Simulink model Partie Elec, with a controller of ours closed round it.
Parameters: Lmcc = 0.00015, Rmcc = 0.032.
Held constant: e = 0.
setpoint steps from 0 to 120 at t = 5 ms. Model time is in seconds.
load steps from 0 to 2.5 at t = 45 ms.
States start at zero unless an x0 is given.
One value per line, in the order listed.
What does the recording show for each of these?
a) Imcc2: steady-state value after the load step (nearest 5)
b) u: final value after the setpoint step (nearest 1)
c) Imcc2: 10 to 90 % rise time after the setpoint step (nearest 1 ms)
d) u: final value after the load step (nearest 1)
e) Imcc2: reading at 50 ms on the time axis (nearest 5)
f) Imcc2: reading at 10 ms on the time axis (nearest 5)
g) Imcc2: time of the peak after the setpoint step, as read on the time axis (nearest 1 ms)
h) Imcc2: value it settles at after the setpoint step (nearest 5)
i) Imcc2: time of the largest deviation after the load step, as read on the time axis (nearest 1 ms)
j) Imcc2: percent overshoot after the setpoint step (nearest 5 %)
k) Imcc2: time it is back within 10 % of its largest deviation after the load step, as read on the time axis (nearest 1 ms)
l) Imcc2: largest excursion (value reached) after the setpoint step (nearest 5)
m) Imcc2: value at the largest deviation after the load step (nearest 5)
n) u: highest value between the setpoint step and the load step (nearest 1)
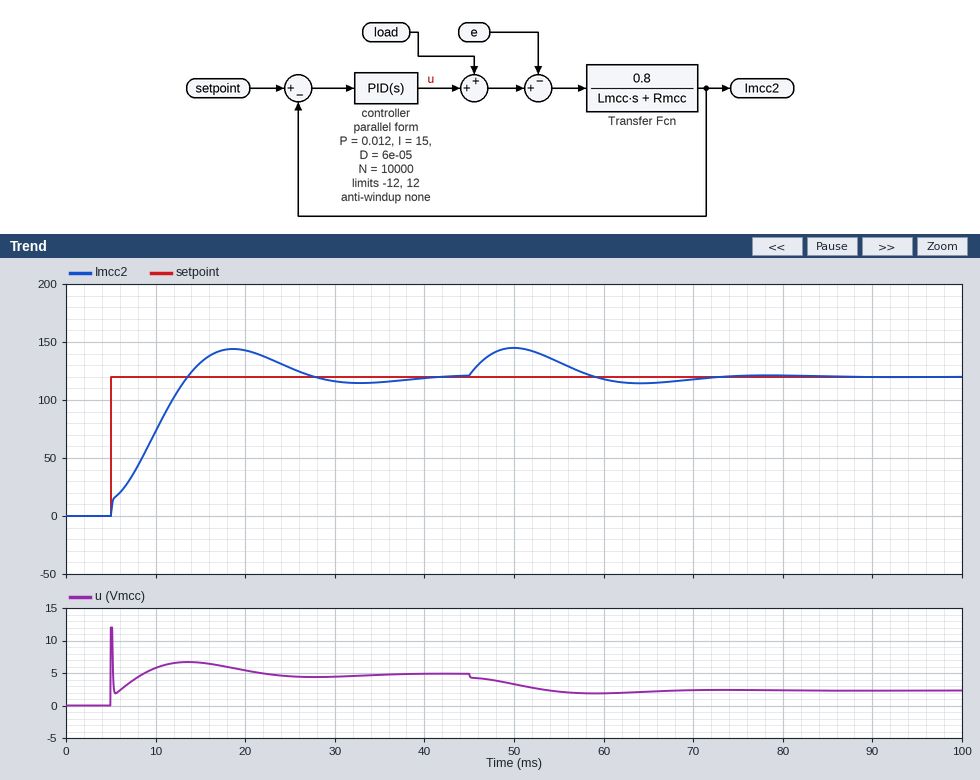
120
5
7 ms
2
145
75
19 ms
120
50 ms
20 %
70 ms
145
145
12
